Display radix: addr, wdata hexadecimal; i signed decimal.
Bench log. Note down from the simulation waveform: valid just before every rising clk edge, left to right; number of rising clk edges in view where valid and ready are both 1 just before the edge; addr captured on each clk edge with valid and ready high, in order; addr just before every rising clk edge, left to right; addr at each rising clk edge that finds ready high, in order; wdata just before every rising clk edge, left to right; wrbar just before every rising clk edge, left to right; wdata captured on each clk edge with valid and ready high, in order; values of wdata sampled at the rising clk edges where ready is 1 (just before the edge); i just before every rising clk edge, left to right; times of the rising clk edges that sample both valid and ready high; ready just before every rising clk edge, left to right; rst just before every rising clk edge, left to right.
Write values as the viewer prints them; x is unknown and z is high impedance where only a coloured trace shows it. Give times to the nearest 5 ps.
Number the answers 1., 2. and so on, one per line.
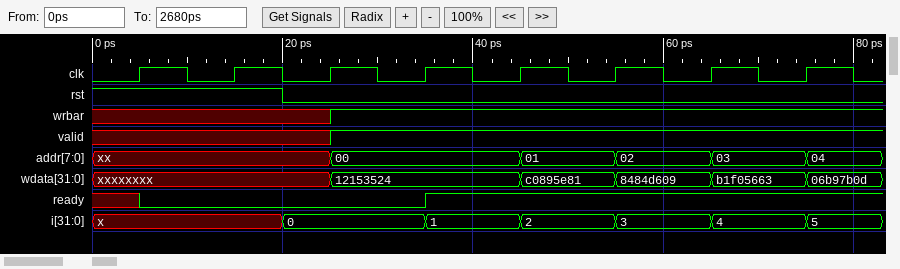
1. x x x 1 1 1 1 1
2. 4
3. 00, 01, 02, 03
4. xx, xx, xx, 00, 00, 01, 02, 03
5. 00, 01, 02, 03
6. xxxxxxxx, xxxxxxxx, xxxxxxxx, 12153524, 12153524, c0895e81, 8484d609, b1f05663
7. x x x 1 1 1 1 1
8. 12153524, c0895e81, 8484d609, b1f05663
9. 12153524, c0895e81, 8484d609, b1f05663
10. x, x, 0, 0, 1, 2, 3, 4
11. 45 ps, 55 ps, 65 ps, 75 ps
12. x 0 0 0 1 1 1 1
13. 1 1 0 0 0 0 0 0
